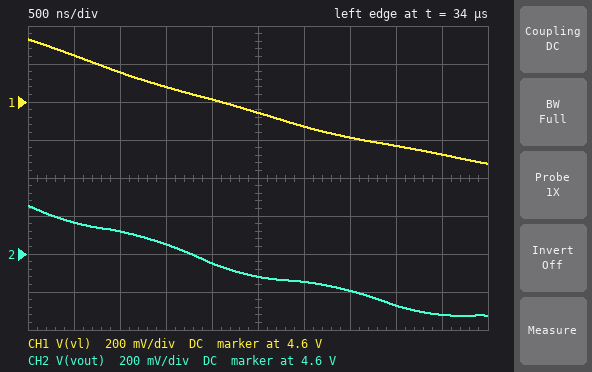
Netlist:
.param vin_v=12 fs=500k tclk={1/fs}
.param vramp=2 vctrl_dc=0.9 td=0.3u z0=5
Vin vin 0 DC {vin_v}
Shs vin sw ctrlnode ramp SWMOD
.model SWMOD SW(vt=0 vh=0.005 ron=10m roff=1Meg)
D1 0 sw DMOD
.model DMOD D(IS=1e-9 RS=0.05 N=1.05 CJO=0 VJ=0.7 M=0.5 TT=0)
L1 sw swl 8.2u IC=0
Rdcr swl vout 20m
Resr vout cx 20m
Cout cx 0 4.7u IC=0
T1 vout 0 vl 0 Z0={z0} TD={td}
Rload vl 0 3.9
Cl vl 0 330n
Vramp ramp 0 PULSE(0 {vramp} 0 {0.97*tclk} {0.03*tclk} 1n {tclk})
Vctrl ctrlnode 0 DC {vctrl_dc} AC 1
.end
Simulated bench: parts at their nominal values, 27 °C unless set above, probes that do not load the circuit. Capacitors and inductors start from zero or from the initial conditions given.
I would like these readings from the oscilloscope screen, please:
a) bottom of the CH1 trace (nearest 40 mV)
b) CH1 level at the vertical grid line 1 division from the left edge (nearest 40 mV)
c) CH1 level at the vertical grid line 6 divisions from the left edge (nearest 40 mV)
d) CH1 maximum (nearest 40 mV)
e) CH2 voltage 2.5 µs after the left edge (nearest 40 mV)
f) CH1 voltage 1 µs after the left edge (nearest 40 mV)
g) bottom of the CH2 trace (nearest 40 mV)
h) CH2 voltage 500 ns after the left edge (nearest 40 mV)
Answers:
4.28 V
4.84 V
4.48 V
4.92 V
4.48 V
4.76 V
4.28 V
4.76 V
